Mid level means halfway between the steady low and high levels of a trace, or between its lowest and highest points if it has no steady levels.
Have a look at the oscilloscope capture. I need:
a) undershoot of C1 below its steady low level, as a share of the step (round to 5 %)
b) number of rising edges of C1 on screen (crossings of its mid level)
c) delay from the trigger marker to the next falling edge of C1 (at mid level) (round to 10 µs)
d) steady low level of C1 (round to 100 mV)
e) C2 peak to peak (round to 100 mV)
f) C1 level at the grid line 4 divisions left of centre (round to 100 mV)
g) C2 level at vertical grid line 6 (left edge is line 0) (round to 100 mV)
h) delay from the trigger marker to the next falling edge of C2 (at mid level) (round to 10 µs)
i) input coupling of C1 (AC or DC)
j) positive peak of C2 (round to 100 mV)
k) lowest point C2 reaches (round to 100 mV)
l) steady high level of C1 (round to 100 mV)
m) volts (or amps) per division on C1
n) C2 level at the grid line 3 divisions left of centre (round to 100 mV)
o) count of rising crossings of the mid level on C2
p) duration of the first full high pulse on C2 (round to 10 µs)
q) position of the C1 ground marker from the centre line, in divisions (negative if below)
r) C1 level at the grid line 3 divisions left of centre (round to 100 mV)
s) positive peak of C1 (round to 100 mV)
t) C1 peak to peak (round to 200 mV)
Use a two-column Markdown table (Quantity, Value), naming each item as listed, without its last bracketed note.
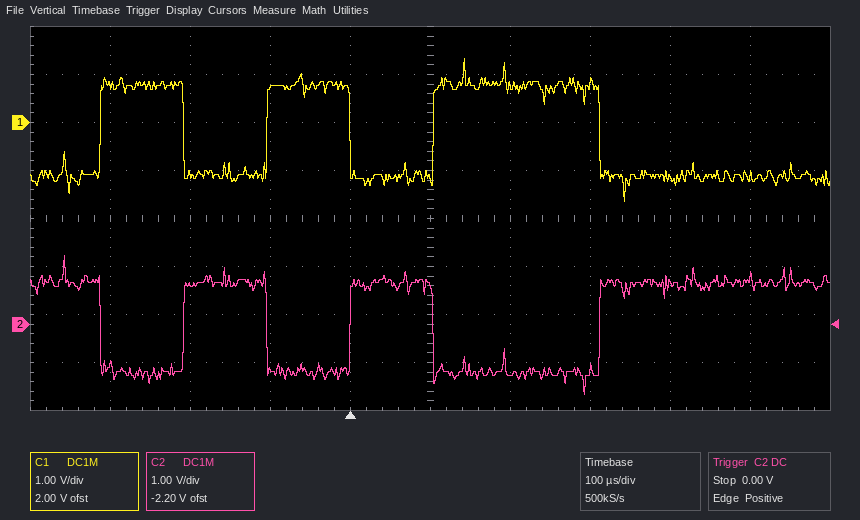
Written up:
| Quantity | Value |
|---|---|
| undershoot of C1 below its steady low level, as a share of the step | 30 % |
| number of rising edges of C1 on screen | 3 |
| delay from the trigger marker to the next falling edge of C1 (at mid level) | 310 µs |
| steady low level of C1 | -1.1 V |
| C2 peak to peak | 2.9 V |
| C1 level at the grid line 4 divisions left of centre | 800 mV |
| C2 level at vertical grid line 6 (left edge is line 0) | -1.0 V |
| delay from the trigger marker to the next falling edge of C2 (at mid level) | 100 µs |
| input coupling of C1 | DC |
| positive peak of C2 | 1.4 V |
| lowest point C2 reaches | -1.5 V |
| steady high level of C1 | 800 mV |
| volts (or amps) per division on C1 | 1 V |
| C2 level at the grid line 3 divisions left of centre | 800 mV |
| count of rising crossings of the mid level on C2 | 3 |
| duration of the first full high pulse on C2 | 100 µs |
| position of the C1 ground marker from the centre line, in divisions | +2.0 div |
| C1 level at the grid line 3 divisions left of centre | -1.1 V |
| positive peak of C1 | 1.3 V |
| C1 peak to peak | 3.0 V |
